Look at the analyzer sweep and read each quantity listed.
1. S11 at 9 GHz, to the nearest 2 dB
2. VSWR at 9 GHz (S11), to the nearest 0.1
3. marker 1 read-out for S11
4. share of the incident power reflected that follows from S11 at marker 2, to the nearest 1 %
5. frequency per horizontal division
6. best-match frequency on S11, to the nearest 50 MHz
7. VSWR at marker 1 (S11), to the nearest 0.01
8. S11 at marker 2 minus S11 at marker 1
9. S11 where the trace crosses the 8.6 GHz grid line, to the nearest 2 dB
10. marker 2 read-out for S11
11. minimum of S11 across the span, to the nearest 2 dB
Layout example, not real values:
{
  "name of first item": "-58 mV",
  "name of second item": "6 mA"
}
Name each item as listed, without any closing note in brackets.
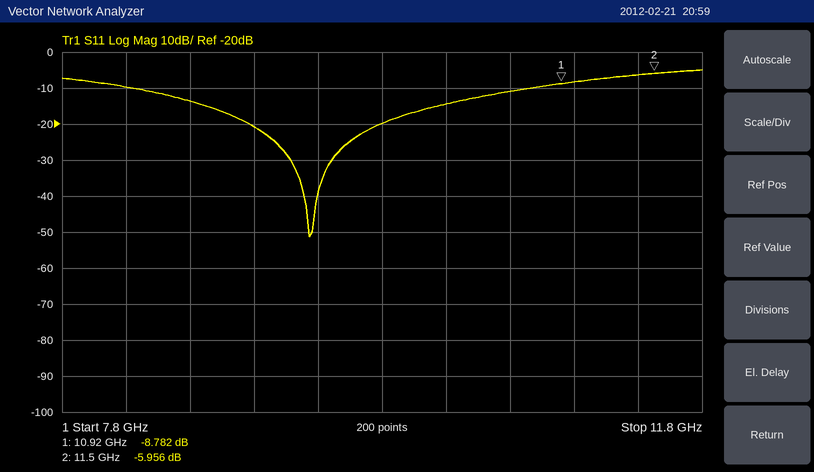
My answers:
{
  "S11 at 9 GHz, to the nearest 2 dB": "-20 dB",
  "VSWR at 9 GHz (S11), to the nearest 0.1": "1.2",
  "marker 1 read-out for S11": "-8.782 dB",
  "share of the incident power reflected that follows from S11 at marker 2, to the nearest 1 %": "25 %",
  "frequency per horizontal division": "400 MHz",
  "best-match frequency on S11, to the nearest 50 MHz": "9.35 GHz",
  "VSWR at marker 1 (S11), to the nearest 0.01": "2.14",
  "S11 at marker 2 minus S11 at marker 1": "2.826 dB",
  "S11 where the trace crosses the 8.6 GHz grid line, to the nearest 2 dB": "-14 dB",
  "marker 2 read-out for S11": "-5.956 dB",
  "minimum of S11 across the span, to the nearest 2 dB": "-52 dB"
}
